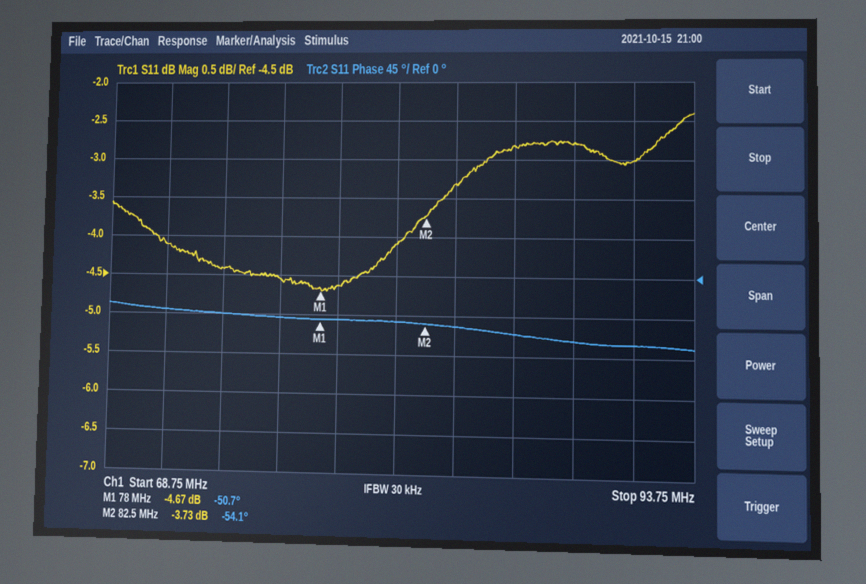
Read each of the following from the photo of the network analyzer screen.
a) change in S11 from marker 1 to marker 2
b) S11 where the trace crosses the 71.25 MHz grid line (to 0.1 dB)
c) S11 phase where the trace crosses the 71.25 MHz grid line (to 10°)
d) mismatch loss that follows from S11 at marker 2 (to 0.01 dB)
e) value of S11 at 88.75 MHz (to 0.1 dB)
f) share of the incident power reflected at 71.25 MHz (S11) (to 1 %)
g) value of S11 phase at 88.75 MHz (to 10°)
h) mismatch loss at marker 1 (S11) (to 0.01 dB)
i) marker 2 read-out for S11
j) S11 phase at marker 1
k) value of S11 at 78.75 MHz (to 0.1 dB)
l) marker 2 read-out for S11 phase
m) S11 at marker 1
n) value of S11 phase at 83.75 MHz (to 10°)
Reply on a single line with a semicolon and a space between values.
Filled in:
0.94 dB; -4.1 dB; -40°; 2.39 dB; -2.8 dB; 39 %; -70°; 1.81 dB; -3.73 dB; -50.7°; -4.6 dB; -54.1°; -4.67 dB; -60°
